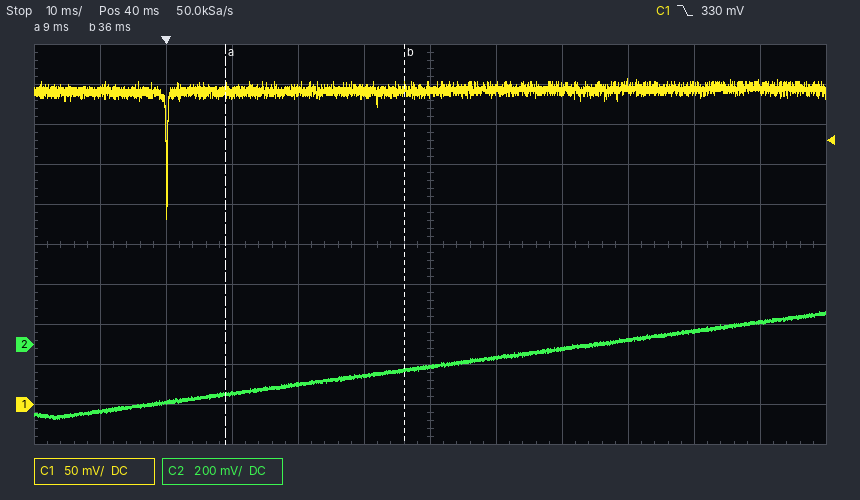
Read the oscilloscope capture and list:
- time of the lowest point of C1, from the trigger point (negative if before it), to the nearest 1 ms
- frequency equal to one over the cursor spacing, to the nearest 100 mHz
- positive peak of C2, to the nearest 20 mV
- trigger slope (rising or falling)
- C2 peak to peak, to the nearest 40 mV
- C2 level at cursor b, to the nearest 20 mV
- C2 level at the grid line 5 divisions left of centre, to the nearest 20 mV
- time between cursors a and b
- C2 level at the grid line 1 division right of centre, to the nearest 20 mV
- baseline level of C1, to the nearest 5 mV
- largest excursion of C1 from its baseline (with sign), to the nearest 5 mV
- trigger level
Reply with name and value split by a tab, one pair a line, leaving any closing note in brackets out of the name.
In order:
time of the lowest point of C1, from the trigger point (negative if before it), to the nearest 1 ms	0 ms
frequency equal to one over the cursor spacing, to the nearest 100 mHz	37.0 Hz
positive peak of C2, to the nearest 20 mV	160 mV
trigger slope	falling
C2 peak to peak, to the nearest 40 mV	520 mV
C2 level at cursor b, to the nearest 20 mV	-120 mV
C2 level at the grid line 5 divisions left of centre, to the nearest 20 mV	-340 mV
time between cursors a and b	27 ms
C2 level at the grid line 1 division right of centre, to the nearest 20 mV	-60 mV
baseline level of C1, to the nearest 5 mV	395 mV
largest excursion of C1 from its baseline (with sign), to the nearest 5 mV	-160 mV
trigger level	330 mV
